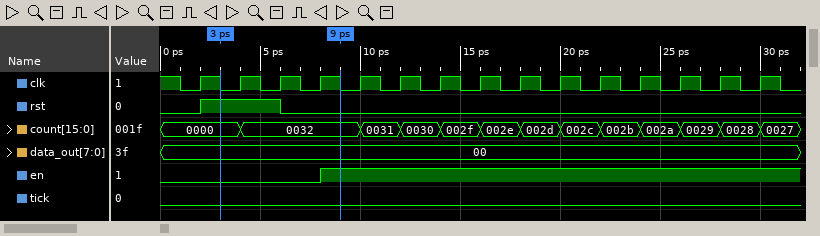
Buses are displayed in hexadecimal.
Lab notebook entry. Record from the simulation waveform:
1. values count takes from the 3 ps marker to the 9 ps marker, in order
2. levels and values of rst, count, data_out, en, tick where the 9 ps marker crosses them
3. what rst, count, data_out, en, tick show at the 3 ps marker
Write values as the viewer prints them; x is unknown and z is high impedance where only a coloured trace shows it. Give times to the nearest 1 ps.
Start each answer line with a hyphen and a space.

- 0000, 0032
- rst=0, count=0032, data_out=00, en=1, tick=0
- rst=1, count=0000, data_out=00, en=0, tick=0
